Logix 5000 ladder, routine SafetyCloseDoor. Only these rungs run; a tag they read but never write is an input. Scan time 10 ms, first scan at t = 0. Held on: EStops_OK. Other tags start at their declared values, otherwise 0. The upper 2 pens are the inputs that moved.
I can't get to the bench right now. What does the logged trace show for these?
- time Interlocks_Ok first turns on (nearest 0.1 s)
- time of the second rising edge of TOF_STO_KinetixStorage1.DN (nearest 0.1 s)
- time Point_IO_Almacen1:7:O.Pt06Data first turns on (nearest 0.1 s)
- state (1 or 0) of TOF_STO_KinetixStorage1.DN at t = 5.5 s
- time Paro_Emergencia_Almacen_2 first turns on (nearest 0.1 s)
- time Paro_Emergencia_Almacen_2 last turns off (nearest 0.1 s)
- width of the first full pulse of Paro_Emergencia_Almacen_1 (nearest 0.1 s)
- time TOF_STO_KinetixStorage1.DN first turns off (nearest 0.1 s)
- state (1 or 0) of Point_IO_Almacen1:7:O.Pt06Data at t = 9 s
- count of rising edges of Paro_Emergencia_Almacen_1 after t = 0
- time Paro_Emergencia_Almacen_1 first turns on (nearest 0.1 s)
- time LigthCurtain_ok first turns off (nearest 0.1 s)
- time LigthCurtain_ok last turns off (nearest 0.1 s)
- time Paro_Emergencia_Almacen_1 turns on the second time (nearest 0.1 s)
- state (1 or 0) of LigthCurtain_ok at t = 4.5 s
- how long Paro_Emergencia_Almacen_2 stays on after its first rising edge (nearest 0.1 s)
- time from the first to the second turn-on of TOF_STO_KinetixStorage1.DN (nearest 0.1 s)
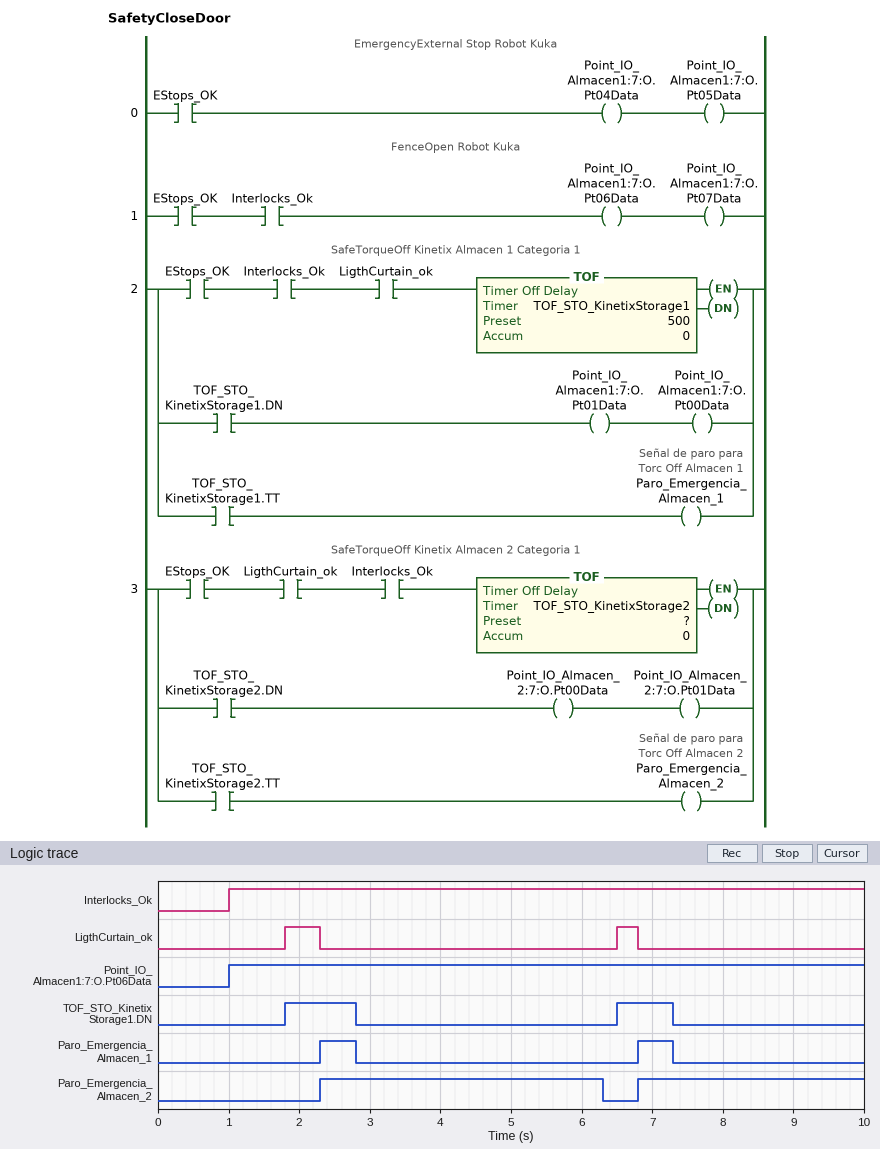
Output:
1.0 s
6.5 s
1.0 s
0
2.3 s
6.3 s
0.5 s
2.8 s
1
2
2.3 s
2.3 s
6.8 s
6.8 s
0
4.0 s
4.7 s
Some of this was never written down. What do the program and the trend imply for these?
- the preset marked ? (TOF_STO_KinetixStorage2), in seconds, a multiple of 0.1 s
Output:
4.0 s
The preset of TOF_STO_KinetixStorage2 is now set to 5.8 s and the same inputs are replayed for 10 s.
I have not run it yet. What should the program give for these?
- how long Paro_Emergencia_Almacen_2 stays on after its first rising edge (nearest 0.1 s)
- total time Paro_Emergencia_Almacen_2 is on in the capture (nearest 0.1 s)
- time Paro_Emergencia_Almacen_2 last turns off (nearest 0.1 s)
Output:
4.2 s
7.4 s
6.5 s
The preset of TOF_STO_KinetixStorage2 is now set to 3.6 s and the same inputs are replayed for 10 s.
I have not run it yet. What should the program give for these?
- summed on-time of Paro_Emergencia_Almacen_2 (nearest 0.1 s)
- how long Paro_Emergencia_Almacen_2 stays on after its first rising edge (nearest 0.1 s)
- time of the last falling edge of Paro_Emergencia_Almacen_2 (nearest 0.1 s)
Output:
6.8 s
3.6 s
5.9 s
